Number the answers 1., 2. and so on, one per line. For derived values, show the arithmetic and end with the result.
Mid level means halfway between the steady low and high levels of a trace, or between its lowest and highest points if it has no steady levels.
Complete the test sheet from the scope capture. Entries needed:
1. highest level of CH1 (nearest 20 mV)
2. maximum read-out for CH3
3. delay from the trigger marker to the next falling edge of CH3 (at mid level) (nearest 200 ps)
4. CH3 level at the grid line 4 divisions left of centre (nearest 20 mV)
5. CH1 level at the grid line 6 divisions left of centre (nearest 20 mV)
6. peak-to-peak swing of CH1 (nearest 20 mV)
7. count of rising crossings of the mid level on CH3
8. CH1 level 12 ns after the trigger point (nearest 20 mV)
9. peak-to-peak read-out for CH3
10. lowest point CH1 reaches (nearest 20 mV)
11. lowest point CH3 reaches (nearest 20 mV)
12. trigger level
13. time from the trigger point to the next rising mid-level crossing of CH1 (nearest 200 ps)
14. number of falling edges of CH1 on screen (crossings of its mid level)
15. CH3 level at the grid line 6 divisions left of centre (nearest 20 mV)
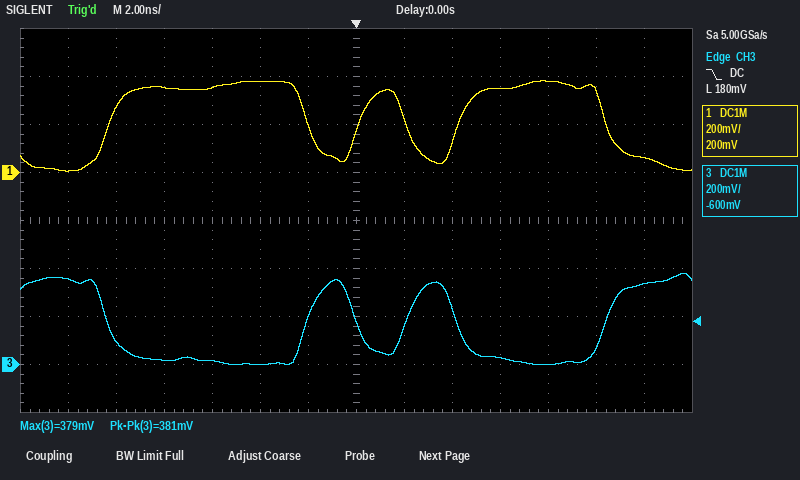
1. 380 mV
2. 379 mV
3. 4.2 ns
4. 20 mV
5. 0 mV
6. 380 mV − (0 mV) = 380 mV
7. 3
8. 60 mV
9. 381 mV
10. 0 mV
11. 0 mV
12. 180 mV
13. 4.2 ns
14. 3
15. 360 mV
